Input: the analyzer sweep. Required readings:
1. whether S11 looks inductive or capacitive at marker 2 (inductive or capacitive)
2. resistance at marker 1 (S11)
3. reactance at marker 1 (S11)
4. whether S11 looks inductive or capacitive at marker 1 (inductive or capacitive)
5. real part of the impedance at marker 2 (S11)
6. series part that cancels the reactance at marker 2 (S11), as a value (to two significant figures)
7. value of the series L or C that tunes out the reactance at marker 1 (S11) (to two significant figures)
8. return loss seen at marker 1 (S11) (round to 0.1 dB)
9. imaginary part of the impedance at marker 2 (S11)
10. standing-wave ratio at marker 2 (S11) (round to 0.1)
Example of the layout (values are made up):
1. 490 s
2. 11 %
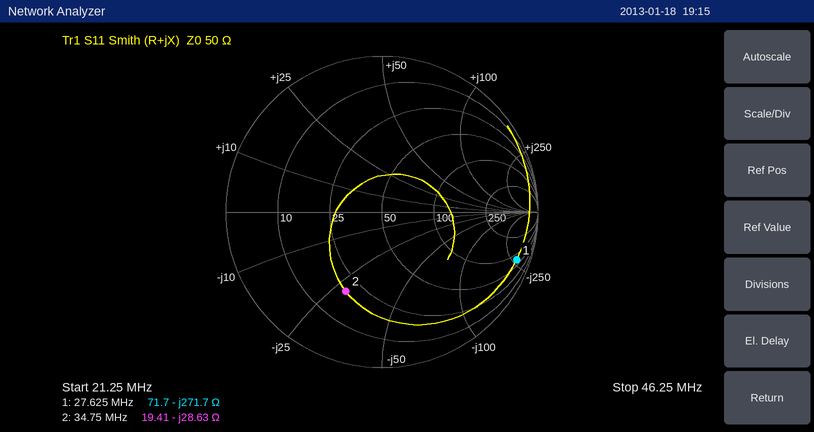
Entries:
1. capacitive
2. 71.7 Ω
3. -271.7 Ω
4. capacitive
5. 19.41 Ω
6. 130 nH
7. 1.6 µH
8. 0.8 dB
9. -28.63 Ω
10. 3.5
